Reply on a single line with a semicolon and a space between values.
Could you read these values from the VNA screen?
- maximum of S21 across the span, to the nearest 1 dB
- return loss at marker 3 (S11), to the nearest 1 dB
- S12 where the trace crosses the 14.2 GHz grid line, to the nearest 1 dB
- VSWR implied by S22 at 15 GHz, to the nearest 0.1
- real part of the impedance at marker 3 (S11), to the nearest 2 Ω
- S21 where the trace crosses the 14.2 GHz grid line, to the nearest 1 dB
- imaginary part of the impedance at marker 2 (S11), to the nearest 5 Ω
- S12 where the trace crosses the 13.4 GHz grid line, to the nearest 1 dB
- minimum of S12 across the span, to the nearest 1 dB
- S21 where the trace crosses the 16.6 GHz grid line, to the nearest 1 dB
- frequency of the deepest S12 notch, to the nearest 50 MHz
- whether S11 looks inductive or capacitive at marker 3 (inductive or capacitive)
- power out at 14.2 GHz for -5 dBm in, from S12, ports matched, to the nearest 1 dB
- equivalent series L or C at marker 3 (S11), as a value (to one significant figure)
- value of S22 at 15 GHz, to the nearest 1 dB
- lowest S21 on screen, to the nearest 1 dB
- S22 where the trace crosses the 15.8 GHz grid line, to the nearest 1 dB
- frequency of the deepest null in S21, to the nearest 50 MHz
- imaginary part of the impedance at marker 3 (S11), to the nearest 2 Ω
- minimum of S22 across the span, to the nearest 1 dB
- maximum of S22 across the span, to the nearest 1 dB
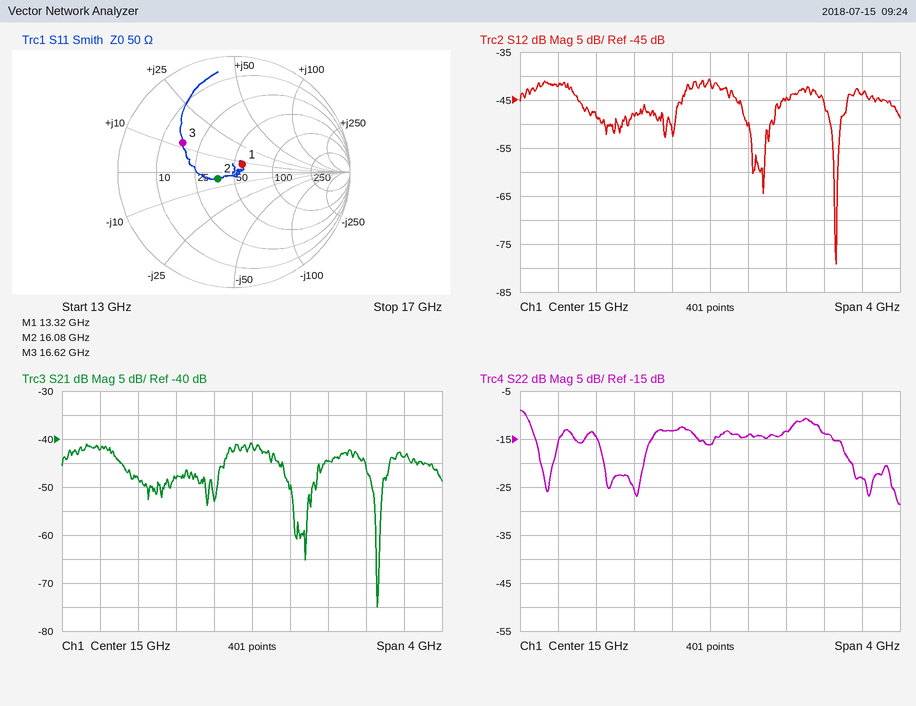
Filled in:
-41 dB; 6 dB; -48 dB; 1.4; 18 Ω; -48 dB; -5 Ω; -42 dB; -79 dB; -44 dB; 16.35 GHz; inductive; -53 dBm; 100 pH; -16 dB; -75 dB; -13 dB; 16.30 GHz; +12 Ω; -29 dB; -9 dB
